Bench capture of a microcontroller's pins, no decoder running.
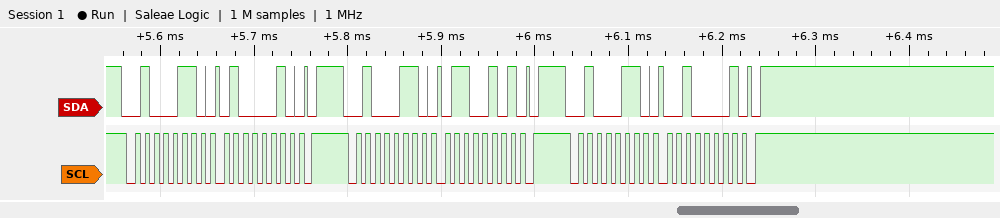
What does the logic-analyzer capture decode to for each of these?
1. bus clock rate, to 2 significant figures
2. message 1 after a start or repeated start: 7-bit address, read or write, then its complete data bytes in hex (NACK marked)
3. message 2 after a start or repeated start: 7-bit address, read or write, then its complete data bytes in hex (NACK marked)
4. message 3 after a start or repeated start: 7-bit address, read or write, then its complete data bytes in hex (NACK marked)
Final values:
100 kHz
0x23 write: 42
0x23 write: 65
0x23 write: 21
